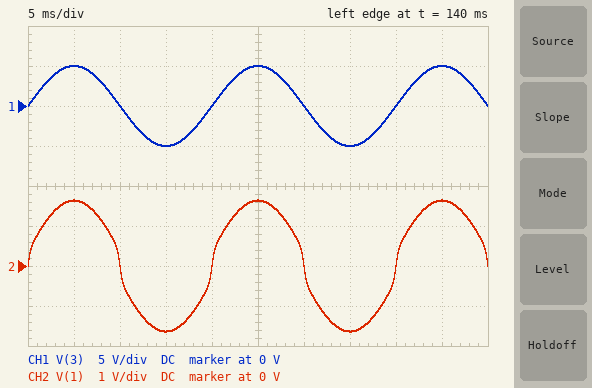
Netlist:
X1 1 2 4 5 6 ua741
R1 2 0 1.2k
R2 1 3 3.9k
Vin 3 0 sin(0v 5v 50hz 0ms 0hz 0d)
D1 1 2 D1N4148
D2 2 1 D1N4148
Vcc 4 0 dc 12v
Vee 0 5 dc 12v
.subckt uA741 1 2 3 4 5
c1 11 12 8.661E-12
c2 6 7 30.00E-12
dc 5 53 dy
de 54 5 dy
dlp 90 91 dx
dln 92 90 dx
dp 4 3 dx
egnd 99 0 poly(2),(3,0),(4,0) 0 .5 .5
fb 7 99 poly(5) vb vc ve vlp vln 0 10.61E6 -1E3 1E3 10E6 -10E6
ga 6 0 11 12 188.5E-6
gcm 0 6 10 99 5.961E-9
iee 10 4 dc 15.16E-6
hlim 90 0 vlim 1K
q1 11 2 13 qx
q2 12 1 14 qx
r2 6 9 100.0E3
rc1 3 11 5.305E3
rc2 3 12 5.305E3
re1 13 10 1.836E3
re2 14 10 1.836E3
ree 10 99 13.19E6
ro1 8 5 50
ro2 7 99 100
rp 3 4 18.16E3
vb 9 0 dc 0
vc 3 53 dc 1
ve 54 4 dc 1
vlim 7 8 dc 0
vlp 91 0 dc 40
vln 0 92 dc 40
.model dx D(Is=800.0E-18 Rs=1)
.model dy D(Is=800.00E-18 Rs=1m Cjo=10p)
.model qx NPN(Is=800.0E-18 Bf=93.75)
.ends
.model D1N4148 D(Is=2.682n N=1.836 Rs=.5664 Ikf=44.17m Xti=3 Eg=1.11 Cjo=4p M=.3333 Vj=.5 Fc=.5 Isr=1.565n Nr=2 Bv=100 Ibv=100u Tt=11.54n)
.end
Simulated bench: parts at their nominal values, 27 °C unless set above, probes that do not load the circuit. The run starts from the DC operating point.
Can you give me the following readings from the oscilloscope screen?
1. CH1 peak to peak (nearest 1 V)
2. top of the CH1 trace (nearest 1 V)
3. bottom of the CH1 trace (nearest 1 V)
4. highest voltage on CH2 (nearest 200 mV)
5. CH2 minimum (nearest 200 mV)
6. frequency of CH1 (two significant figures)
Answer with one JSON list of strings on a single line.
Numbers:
["10 V", "5 V", "-5 V", "1.6 V", "-1.6 V", "50 Hz"]
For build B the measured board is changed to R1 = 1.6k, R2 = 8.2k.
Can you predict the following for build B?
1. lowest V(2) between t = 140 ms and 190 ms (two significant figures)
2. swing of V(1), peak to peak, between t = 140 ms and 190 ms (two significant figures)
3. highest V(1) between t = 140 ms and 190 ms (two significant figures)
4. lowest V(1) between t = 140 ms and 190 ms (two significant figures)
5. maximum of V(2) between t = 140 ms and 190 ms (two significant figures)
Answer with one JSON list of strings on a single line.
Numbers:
["-720 mV", "2.6 V", "1.3 V", "-1.3 V", "720 mV"]
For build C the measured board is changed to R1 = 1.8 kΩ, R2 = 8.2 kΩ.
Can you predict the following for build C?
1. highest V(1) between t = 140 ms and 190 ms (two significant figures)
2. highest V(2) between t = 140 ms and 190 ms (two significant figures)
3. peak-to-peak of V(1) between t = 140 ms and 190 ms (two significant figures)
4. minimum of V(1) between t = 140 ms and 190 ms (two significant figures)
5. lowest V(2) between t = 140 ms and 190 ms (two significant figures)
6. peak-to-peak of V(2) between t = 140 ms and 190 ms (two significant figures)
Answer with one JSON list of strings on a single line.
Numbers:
["1.4 V", "800 mV", "2.7 V", "-1.4 V", "-800 mV", "1.6 V"]
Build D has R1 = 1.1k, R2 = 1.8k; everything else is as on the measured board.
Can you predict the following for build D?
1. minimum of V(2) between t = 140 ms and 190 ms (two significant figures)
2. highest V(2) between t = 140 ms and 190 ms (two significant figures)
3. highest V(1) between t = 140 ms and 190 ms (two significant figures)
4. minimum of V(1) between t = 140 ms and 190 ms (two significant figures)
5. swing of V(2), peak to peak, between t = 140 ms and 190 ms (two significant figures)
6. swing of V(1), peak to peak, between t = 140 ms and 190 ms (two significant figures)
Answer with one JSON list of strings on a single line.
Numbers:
["-1.7 V", "1.7 V", "2.3 V", "-2.3 V", "3.3 V", "4.6 V"]
